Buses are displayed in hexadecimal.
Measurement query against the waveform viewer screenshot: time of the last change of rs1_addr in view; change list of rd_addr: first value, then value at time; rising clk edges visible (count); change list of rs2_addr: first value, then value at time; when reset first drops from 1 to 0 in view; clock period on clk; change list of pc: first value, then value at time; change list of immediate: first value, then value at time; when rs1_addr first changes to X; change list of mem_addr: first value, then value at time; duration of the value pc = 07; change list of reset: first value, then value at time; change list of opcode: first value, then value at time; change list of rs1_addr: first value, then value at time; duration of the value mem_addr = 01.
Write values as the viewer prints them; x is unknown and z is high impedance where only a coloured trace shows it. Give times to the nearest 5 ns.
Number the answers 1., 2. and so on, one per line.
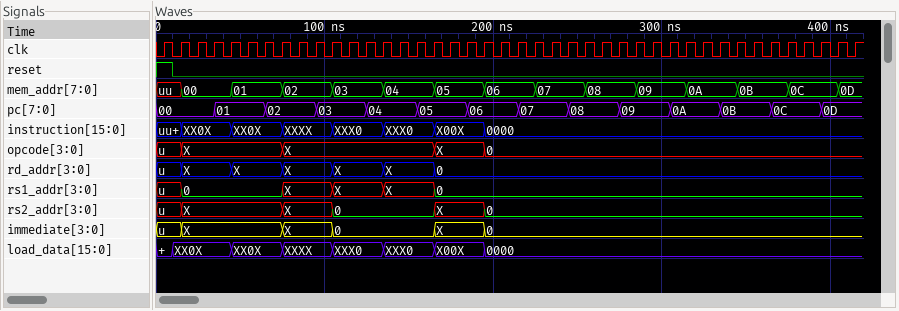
1. 165 ns
2. u, X at 15 ns, X at 45 ns, X at 75 ns, X at 105 ns, X at 135 ns, 0 at 165 ns
3. 42
4. u, X at 15 ns, X at 75 ns, 0 at 105 ns, X at 165 ns, 0 at 195 ns
5. 10 ns
6. 10 ns
7. 00, 01 at 35 ns, 02 at 65 ns, 03 at 95 ns, 04 at 125 ns, 05 at 155 ns, 06 at 185 ns, 07 at 215 ns, 08 at 245 ns, 09 at 275 ns, 0A at 305 ns, 0B at 335 ns, 0C at 365 ns, 0D at 395 ns
8. u, X at 15 ns, X at 75 ns, 0 at 105 ns, X at 165 ns, 0 at 195 ns
9. 75 ns
10. uu, 00 at 15 ns, 01 at 45 ns, 02 at 75 ns, 03 at 105 ns, 04 at 135 ns, 05 at 165 ns, 06 at 195 ns, 07 at 225 ns, 08 at 255 ns, 09 at 285 ns, 0A at 315 ns, 0B at 345 ns, 0C at 375 ns, 0D at 405 ns
11. 30 ns
12. 1, 0 at 10 ns
13. u, X at 15 ns, X at 75 ns, X at 165 ns, 0 at 195 ns
14. u, 0 at 15 ns, X at 75 ns, X at 105 ns, X at 135 ns, 0 at 165 ns
15. 30 ns
